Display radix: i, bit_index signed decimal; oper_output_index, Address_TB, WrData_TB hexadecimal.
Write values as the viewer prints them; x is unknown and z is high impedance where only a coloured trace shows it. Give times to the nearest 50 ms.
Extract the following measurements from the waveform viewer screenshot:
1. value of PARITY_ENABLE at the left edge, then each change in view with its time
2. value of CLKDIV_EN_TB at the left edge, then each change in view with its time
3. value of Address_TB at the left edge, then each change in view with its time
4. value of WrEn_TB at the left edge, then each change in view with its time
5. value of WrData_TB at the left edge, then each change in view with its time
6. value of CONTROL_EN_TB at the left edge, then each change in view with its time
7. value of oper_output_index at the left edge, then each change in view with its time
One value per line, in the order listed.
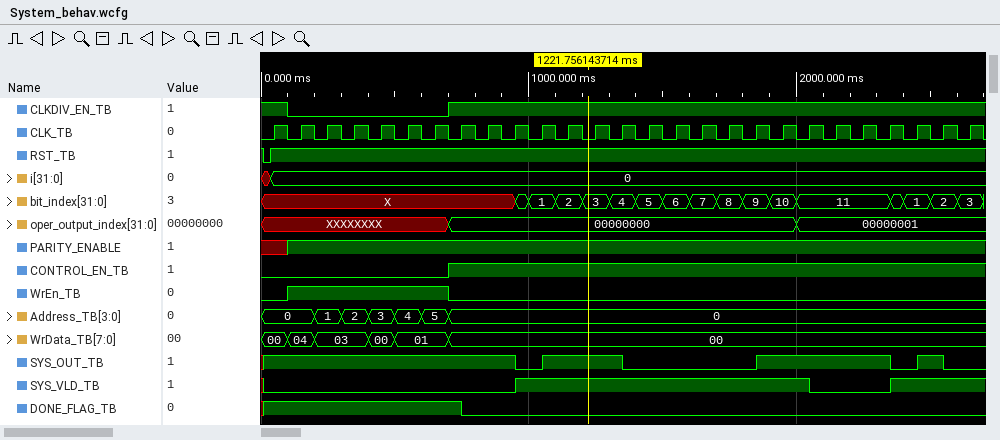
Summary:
x, 1 at 100 ms
1, 0 at 100 ms, 1 at 700 ms
0, 1 at 200 ms, 2 at 300 ms, 3 at 400 ms, 4 at 500 ms, 5 at 600 ms, 0 at 700 ms
0, 1 at 100 ms, 0 at 700 ms
00, 04 at 100 ms, 03 at 200 ms, 00 at 400 ms, 01 at 500 ms, 00 at 700 ms
0, 1 at 700 ms
XXXXXXXX, 00000000 at 700 ms, 00000001 at 2000 ms
